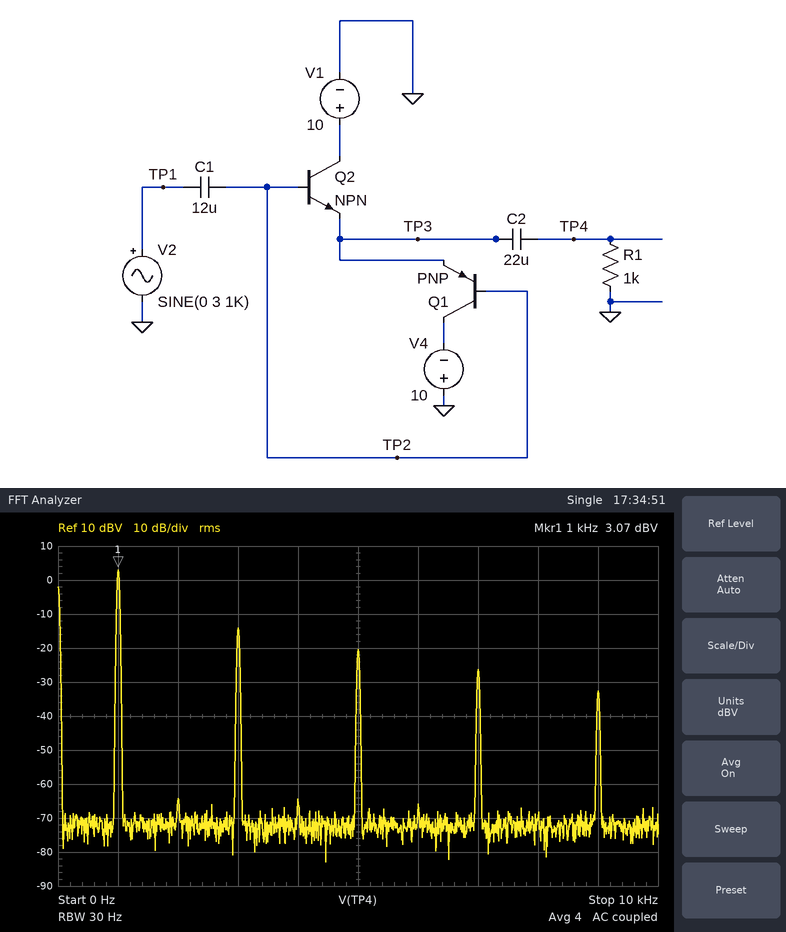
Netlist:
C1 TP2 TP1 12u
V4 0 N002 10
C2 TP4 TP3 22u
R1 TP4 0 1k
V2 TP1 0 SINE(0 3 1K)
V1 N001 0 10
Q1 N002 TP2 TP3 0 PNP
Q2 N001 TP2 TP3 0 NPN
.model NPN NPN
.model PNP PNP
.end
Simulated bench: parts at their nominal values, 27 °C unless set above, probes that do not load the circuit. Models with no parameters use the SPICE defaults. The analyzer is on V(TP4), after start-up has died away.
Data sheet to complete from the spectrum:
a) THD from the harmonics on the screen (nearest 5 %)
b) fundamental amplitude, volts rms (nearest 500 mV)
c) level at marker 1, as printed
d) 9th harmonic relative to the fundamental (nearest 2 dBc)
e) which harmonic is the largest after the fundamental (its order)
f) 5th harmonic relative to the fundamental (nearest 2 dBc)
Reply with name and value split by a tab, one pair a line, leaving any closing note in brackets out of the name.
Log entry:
THD from the harmonics on the screen	15 %
fundamental amplitude, volts rms	1.5 V
level at marker 1, as printed	3.07 dBV
9th harmonic relative to the fundamental	-36 dBc
which harmonic is the largest after the fundamental	3
5th harmonic relative to the fundamental	-24 dBc
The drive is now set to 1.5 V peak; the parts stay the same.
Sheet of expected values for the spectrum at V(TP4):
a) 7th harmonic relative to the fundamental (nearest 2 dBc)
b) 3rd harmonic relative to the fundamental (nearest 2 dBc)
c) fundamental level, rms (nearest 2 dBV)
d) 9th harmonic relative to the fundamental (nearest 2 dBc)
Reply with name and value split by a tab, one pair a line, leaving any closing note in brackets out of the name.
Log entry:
7th harmonic relative to the fundamental	-38 dBc
3rd harmonic relative to the fundamental	-10 dBc
fundamental level, rms	-8 dBV
9th harmonic relative to the fundamental	-32 dBc
